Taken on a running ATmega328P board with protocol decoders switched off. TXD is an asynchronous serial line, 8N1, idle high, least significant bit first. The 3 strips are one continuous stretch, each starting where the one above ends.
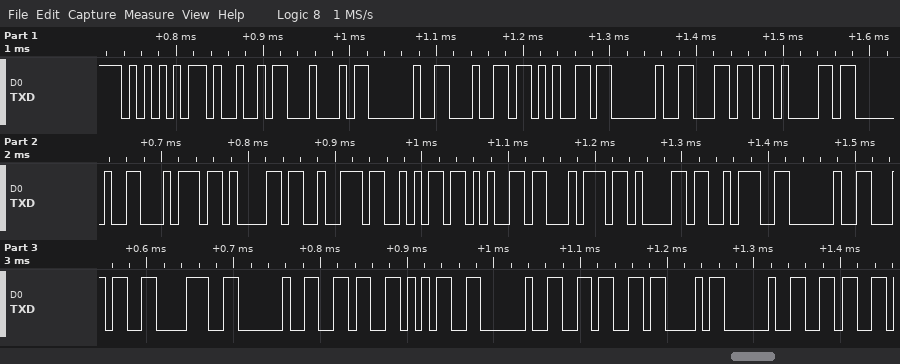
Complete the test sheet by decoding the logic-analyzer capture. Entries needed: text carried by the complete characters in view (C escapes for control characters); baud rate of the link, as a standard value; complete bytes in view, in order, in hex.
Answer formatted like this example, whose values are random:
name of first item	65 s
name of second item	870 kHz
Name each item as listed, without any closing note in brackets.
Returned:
text carried by the complete characters in view	"UID de la tarjeta: 48 65 6C 6"
baud rate of the link, as a standard value	115200 baud
complete bytes in view, in order, in hex	55 49 44 20 64 65 20 6C 61 20 74 61 72 6A 65 74 61 3A 20 34 38 20 36 35 20 36 43 20 36
